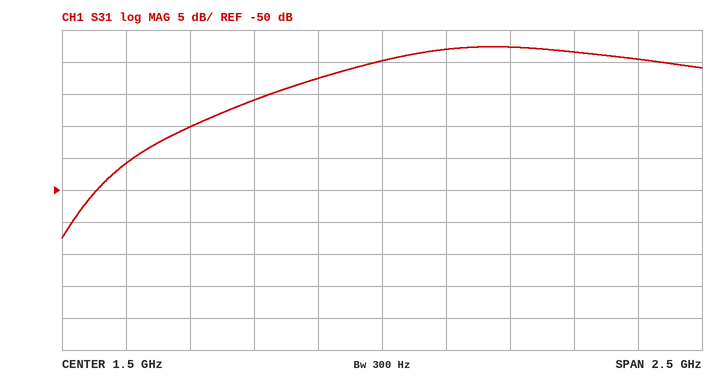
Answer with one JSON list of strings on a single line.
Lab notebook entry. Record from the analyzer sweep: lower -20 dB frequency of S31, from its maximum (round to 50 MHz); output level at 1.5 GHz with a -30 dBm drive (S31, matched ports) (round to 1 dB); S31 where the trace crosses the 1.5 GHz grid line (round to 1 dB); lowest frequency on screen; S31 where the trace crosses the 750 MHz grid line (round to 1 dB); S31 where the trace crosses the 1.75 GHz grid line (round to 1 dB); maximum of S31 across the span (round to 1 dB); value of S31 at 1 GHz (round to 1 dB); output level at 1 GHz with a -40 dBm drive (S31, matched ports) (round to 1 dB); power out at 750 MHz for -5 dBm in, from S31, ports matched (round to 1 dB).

["450 MHz", "-60 dBm", "-30 dB", "250 MHz", "-40 dB", "-28 dB", "-28 dB", "-36 dB", "-76 dBm", "-45 dBm"]
